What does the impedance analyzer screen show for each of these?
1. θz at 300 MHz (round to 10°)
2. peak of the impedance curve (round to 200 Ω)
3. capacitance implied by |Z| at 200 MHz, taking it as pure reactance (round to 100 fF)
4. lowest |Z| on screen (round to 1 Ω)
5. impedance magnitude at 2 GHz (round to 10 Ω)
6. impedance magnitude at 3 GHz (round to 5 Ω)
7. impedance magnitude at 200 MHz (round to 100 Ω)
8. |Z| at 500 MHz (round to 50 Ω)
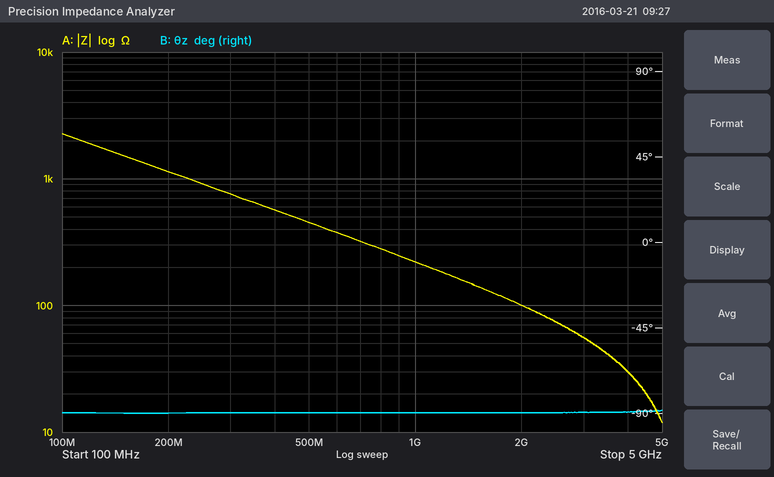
-90°
2.2 kΩ
700 fF
12 Ω
100 Ω
55 Ω
1.1 kΩ
450 Ω
